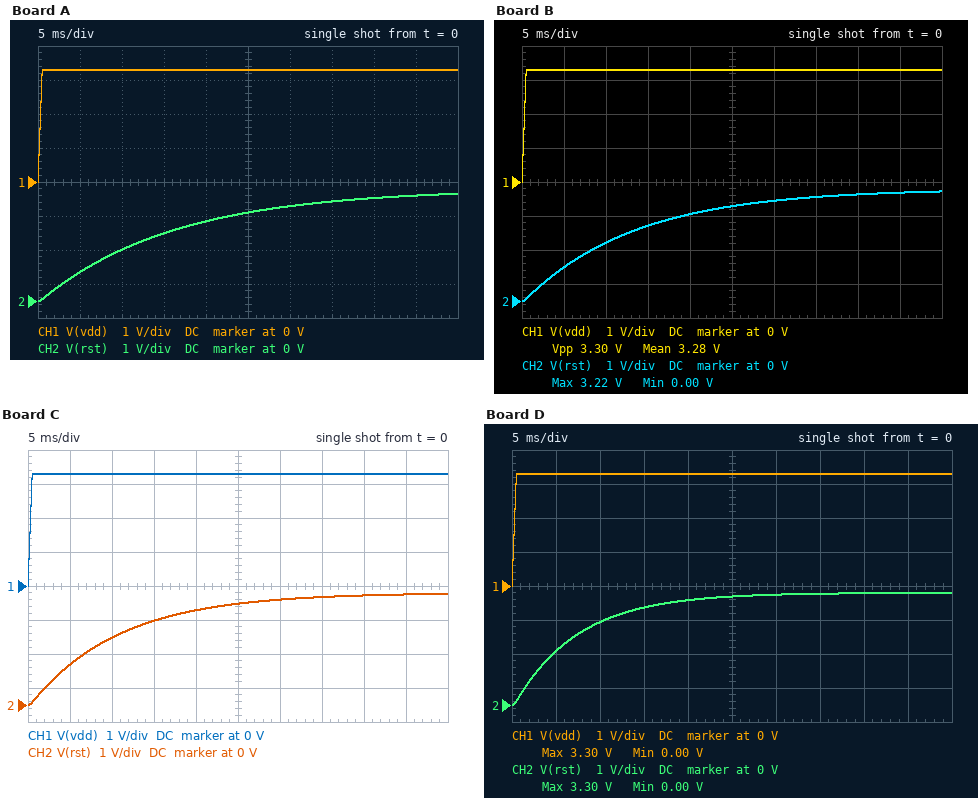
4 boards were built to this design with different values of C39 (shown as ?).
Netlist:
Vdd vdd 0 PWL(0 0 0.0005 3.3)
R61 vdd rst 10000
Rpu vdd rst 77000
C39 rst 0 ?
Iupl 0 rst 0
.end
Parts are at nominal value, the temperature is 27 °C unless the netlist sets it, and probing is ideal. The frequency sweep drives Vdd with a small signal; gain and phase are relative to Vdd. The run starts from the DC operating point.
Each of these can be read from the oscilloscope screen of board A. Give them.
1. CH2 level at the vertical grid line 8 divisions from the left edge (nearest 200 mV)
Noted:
3.0 V
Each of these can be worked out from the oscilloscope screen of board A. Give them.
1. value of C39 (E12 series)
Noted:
1.8 µF
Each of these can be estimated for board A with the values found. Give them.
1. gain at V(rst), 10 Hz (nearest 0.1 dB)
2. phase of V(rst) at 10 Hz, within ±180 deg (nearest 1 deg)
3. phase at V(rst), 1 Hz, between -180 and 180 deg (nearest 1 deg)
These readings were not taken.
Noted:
-3.0 dB
-45 deg
-6 deg
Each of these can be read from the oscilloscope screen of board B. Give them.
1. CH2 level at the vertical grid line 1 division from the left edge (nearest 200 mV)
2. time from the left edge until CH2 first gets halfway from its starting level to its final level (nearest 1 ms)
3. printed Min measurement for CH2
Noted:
1.0 V
9 ms
0.00 V
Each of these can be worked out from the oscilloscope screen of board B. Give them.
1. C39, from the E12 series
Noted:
1.5 µF
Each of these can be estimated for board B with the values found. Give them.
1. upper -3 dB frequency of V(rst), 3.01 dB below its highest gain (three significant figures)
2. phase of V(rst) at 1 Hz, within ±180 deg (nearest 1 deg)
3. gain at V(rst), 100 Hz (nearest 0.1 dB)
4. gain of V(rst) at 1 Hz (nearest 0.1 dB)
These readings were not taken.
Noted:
12.0 Hz
-5 deg
-18.5 dB
0 dB
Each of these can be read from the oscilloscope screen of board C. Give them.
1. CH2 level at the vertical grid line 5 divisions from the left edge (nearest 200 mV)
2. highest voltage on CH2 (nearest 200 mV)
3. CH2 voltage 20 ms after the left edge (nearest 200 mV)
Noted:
3.0 V
3.2 V
2.8 V
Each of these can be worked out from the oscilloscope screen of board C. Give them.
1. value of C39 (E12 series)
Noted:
1.2 µF
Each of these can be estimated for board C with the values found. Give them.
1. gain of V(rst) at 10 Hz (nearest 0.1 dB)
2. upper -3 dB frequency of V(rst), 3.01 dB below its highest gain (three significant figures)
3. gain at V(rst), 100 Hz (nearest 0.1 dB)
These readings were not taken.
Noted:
-1.6 dB
15.0 Hz
-16.6 dB
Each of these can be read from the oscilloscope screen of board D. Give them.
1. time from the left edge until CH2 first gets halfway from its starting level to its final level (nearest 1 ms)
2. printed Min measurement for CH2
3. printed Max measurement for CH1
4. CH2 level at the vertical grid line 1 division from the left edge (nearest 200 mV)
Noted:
5 ms
0.00 V
3.30 V
1.6 V
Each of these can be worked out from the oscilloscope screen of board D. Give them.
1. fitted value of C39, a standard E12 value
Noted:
820 nF
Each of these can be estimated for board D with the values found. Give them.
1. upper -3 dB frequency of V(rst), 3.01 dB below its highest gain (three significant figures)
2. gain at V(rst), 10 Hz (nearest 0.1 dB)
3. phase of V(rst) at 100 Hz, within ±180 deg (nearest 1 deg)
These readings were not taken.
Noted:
21.9 Hz
-0.8 dB
-78 deg
